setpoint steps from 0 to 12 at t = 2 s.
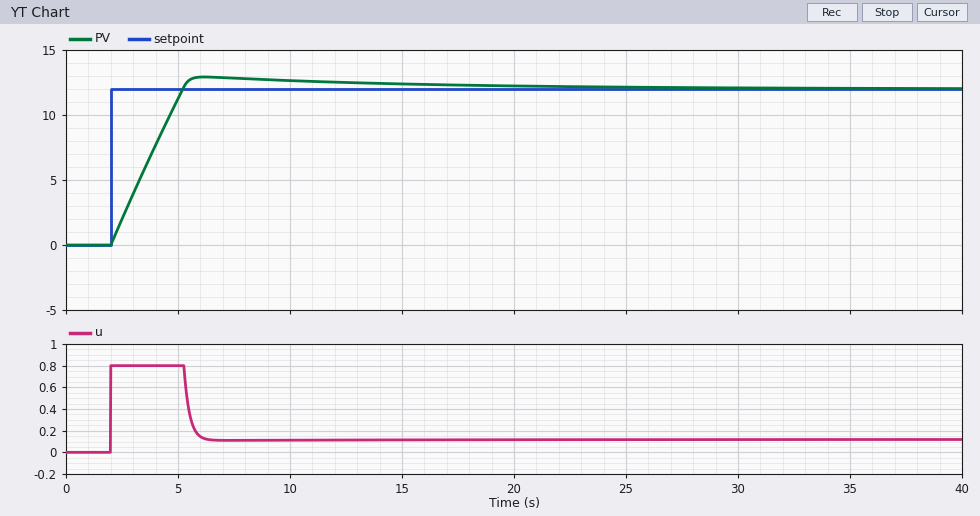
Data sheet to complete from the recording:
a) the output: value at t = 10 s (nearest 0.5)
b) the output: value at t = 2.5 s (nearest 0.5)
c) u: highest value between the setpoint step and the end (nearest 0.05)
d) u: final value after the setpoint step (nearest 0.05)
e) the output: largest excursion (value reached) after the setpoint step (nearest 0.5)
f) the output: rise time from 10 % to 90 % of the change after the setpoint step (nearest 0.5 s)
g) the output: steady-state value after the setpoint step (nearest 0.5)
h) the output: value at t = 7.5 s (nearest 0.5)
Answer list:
12.5
2.0
0.80
0.10
13.0
2.5 s
12.0
13.0
